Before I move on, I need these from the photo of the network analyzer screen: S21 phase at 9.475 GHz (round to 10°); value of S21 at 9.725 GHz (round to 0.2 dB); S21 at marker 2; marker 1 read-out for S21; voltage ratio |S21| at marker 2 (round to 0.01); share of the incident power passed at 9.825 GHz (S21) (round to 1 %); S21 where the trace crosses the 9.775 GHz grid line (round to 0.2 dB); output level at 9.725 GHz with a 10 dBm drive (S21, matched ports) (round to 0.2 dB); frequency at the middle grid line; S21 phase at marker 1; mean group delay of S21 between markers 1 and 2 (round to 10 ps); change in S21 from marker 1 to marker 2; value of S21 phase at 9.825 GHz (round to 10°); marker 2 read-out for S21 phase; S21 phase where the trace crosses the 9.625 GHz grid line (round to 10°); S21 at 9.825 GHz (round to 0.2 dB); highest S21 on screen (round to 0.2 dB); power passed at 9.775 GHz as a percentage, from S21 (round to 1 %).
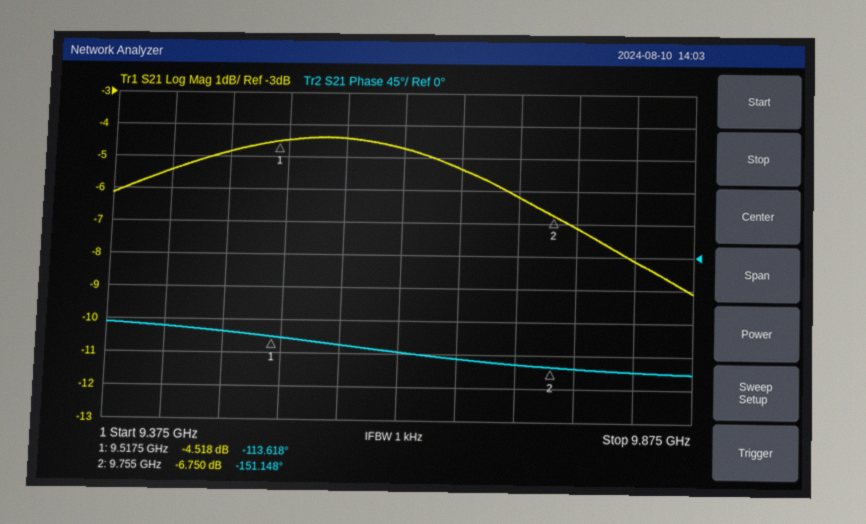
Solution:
-110°
-6.2 dB
-6.750 dB
-4.518 dB
0.46
15 %
-7.2 dB
3.8 dBm
9.625 GHz
-113.618°
440 ps
-2.232 dB
-160°
-151.148°
-130°
-8.2 dB
-4.4 dB
19 %
